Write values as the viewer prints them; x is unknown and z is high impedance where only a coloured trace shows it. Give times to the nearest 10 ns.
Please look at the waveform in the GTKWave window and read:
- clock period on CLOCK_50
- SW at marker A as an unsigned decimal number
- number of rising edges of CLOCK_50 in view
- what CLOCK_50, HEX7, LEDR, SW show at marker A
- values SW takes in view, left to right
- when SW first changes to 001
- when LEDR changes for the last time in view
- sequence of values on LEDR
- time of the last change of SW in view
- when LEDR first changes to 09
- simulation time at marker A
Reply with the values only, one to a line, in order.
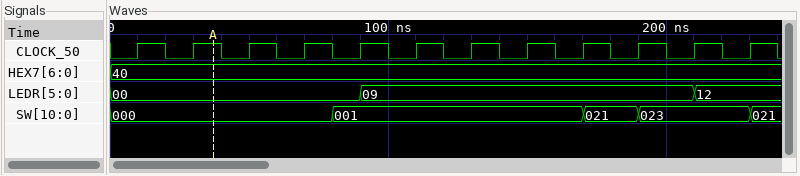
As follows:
20 ns
0
12
CLOCK_50=1, HEX7=40, LEDR=00, SW=000
000, 001, 021, 023, 021
80 ns
210 ns
00, 09, 12
230 ns
90 ns
40 ns
